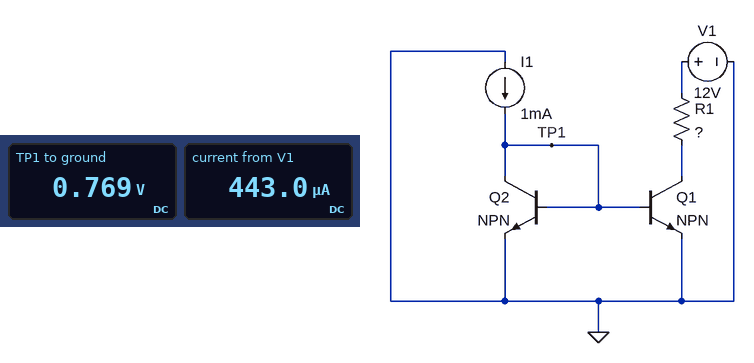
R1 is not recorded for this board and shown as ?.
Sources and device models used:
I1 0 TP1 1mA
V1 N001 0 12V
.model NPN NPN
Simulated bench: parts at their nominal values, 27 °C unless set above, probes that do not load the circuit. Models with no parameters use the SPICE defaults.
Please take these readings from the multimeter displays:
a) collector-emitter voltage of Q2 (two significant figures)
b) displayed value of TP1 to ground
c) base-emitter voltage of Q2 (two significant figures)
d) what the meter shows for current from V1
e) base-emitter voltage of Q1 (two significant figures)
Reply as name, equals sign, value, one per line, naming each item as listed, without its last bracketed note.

collector-emitter voltage of Q2 = 770 mV
displayed value of TP1 to ground = 0.769 V
base-emitter voltage of Q2 = 770 mV
what the meter shows for current from V1 = 443.0 µA
base-emitter voltage of Q1 = 770 mV
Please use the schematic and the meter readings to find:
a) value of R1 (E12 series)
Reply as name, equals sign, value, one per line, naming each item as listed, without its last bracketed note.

value of R1 = 27 kΩ
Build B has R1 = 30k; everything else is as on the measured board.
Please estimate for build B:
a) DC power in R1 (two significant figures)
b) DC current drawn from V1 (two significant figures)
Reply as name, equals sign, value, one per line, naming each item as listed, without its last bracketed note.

DC power in R1 = 4.8 mW
DC current drawn from V1 = 400 µA
